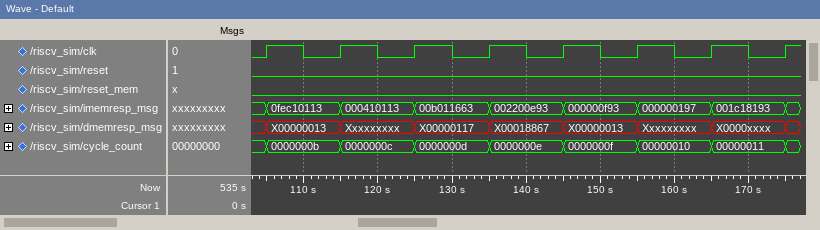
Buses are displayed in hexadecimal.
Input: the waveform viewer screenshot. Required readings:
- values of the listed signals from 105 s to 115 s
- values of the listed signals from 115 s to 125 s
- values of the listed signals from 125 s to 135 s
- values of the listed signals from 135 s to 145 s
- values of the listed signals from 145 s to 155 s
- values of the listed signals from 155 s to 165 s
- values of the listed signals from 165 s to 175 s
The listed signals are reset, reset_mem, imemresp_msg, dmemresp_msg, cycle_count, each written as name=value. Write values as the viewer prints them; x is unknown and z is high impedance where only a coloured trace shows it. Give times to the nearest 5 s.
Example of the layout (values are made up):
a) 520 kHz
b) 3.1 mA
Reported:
a) reset=0, reset_mem=0, imemresp_msg=0fec10113, dmemresp_msg=X00000013, cycle_count=0000000b
b) reset=0, reset_mem=0, imemresp_msg=000410113, dmemresp_msg=Xxxxxxxxx, cycle_count=0000000c
c) reset=0, reset_mem=0, imemresp_msg=00b011663, dmemresp_msg=X00000117, cycle_count=0000000d
d) reset=0, reset_mem=0, imemresp_msg=002200e93, dmemresp_msg=X00018867, cycle_count=0000000e
e) reset=0, reset_mem=0, imemresp_msg=000000f93, dmemresp_msg=X00000013, cycle_count=0000000f
f) reset=0, reset_mem=0, imemresp_msg=000000197, dmemresp_msg=Xxxxxxxxx, cycle_count=00000010
g) reset=0, reset_mem=0, imemresp_msg=001c18193, dmemresp_msg=X0000xxxx, cycle_count=00000011
